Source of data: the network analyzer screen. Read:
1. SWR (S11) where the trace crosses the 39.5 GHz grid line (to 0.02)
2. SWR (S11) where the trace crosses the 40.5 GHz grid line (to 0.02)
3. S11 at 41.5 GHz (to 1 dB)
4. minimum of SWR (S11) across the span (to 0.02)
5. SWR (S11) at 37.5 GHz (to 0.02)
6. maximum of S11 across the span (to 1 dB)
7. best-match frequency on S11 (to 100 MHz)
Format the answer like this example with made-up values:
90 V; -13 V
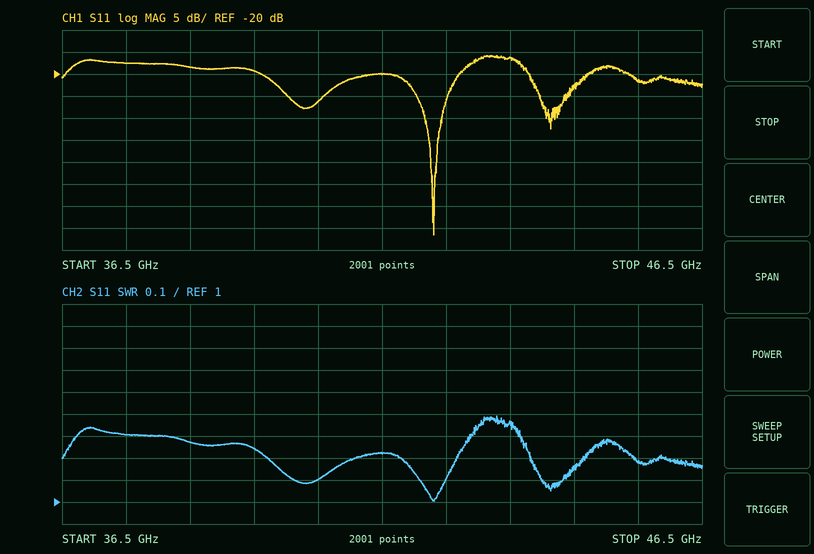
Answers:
1.24; 1.10; -20 dB; 1.00; 1.30; -16 dB; 42.3 GHz
